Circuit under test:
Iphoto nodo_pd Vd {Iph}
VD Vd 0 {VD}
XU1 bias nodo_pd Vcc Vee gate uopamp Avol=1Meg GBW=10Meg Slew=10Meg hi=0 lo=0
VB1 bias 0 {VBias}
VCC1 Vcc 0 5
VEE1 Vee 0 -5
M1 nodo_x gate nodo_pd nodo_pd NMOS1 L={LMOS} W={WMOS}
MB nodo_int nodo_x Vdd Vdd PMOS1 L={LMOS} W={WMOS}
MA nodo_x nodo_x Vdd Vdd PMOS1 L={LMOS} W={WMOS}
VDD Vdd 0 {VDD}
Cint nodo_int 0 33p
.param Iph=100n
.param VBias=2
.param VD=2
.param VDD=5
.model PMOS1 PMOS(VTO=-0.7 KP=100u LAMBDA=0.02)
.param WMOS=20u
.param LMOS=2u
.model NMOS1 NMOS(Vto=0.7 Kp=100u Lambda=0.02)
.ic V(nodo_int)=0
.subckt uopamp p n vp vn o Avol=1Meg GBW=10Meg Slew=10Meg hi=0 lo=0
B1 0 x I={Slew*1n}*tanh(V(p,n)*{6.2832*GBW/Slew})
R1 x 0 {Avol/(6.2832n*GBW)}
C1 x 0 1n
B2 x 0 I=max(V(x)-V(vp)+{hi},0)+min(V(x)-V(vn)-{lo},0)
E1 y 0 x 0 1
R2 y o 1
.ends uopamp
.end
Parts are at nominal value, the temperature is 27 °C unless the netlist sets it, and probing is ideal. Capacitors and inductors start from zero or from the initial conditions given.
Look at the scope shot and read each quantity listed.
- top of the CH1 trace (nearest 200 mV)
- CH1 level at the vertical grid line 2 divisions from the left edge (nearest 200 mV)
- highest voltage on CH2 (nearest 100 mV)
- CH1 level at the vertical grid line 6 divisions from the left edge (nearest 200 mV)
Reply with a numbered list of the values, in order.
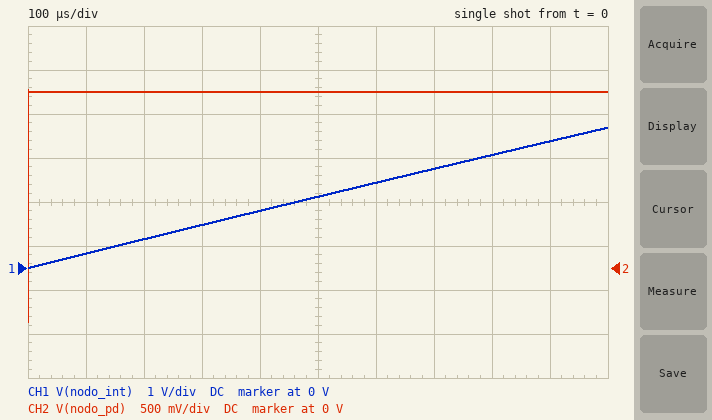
1. 3.2 V
2. 600 mV
3. 2.0 V
4. 2.0 V
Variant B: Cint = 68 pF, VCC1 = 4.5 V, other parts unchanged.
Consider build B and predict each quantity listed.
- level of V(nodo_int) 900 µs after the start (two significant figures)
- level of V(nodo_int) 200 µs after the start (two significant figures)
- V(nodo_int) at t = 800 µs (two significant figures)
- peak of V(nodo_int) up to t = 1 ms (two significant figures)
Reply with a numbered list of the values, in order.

1. 1.4 V
2. 320 mV
3. 1.3 V
4. 1.6 V
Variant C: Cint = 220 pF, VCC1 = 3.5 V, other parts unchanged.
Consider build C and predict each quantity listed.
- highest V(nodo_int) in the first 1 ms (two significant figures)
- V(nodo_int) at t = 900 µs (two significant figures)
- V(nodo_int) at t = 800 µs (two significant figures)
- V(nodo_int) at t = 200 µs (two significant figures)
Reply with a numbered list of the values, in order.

1. 490 mV
2. 440 mV
3. 390 mV
4. 99 mV
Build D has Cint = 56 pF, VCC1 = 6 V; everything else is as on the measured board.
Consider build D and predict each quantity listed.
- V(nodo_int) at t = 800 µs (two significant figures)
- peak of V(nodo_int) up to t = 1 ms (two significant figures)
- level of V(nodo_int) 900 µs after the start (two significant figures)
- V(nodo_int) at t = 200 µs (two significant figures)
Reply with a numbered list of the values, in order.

1. 1.5 V
2. 1.9 V
3. 1.7 V
4. 390 mV
